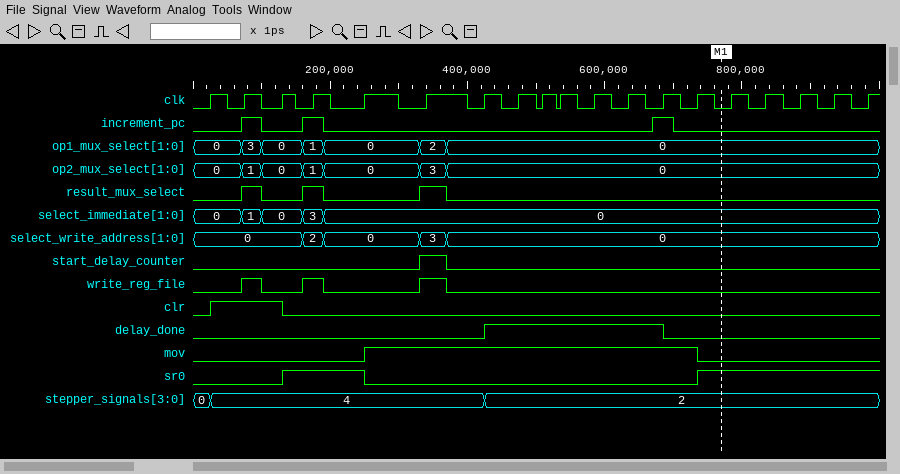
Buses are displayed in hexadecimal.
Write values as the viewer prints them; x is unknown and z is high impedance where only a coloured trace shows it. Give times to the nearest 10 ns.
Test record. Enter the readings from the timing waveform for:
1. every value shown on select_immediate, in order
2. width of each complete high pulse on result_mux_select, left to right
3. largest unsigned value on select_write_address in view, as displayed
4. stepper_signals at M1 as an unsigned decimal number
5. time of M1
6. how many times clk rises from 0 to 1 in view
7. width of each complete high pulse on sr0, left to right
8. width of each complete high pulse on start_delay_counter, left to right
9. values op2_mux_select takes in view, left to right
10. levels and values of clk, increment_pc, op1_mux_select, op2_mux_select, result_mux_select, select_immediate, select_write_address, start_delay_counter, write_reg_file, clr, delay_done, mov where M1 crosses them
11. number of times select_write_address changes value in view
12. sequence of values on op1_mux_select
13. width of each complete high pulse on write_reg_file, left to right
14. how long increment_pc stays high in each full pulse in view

0, 1, 0, 3, 0
30 ns, 30 ns, 40 ns
3
2
770 ns
19
120 ns
40 ns
0, 1, 0, 1, 0, 3, 0
clk=0, increment_pc=0, op1_mux_select=0, op2_mux_select=0, result_mux_select=0, select_immediate=0, select_write_address=0, start_delay_counter=0, write_reg_file=0, clr=0, delay_done=0, mov=0
4
0, 3, 0, 1, 0, 2, 0
30 ns, 30 ns, 40 ns
30 ns, 30 ns, 30 ns
